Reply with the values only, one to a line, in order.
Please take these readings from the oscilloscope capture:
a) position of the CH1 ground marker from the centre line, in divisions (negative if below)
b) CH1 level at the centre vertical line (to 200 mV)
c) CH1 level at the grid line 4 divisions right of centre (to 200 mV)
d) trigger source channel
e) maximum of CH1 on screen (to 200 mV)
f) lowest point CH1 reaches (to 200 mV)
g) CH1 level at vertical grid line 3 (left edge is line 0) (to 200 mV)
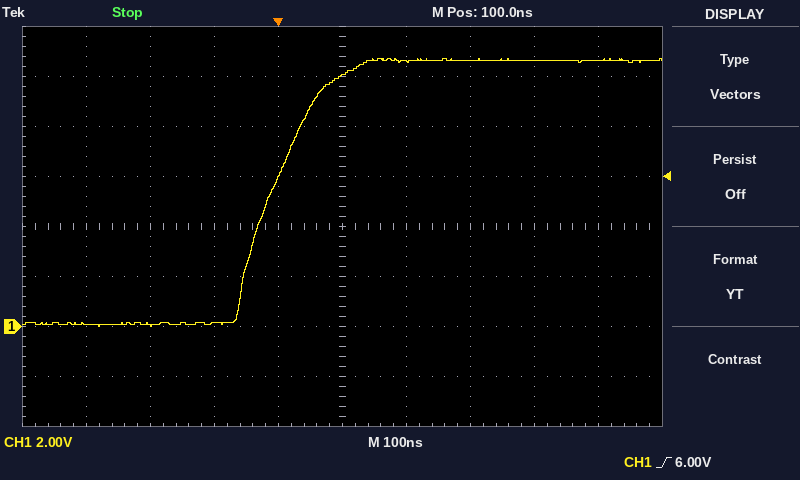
-2.0 div
10.0 V
10.6 V
CH1
10.8 V
0.0 V
200 mV
